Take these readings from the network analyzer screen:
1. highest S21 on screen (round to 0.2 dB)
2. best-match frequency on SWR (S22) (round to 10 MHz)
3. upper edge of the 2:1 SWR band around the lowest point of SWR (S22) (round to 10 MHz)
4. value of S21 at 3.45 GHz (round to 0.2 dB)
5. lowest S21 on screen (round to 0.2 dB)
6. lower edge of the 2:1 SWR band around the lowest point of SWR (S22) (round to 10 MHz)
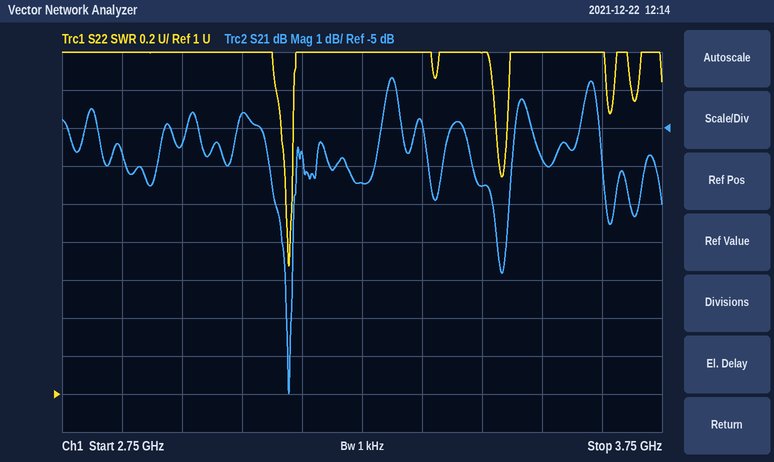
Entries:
-3.6 dB
3.13 GHz
3.13 GHz
-6.6 dB
-12.0 dB
3.12 GHz
